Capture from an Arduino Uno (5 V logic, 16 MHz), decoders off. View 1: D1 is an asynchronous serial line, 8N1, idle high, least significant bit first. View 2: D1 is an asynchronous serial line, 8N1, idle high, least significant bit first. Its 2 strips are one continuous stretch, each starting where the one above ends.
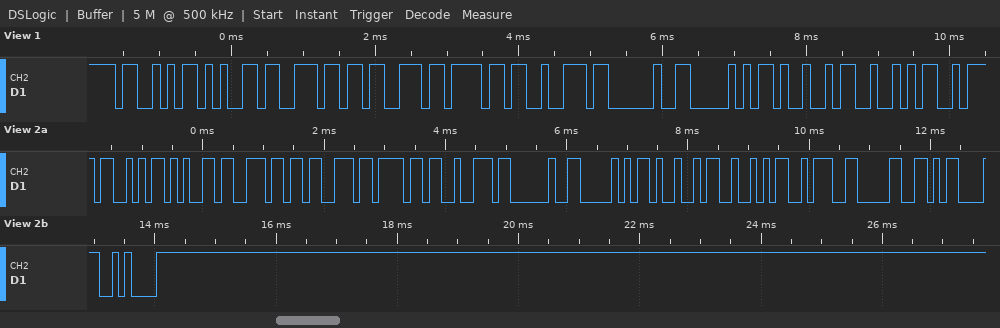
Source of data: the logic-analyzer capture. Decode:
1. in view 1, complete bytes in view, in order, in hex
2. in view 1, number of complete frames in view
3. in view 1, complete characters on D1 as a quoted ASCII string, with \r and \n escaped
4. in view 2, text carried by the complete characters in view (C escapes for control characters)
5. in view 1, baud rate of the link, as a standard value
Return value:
0x53 0x65 0x6E 0x73 0x6F 0x72 0x20 0x50 0x49 0x52
10
"Sensor PIR"
"Sensor PIR:0\r\n"
9600 baud
